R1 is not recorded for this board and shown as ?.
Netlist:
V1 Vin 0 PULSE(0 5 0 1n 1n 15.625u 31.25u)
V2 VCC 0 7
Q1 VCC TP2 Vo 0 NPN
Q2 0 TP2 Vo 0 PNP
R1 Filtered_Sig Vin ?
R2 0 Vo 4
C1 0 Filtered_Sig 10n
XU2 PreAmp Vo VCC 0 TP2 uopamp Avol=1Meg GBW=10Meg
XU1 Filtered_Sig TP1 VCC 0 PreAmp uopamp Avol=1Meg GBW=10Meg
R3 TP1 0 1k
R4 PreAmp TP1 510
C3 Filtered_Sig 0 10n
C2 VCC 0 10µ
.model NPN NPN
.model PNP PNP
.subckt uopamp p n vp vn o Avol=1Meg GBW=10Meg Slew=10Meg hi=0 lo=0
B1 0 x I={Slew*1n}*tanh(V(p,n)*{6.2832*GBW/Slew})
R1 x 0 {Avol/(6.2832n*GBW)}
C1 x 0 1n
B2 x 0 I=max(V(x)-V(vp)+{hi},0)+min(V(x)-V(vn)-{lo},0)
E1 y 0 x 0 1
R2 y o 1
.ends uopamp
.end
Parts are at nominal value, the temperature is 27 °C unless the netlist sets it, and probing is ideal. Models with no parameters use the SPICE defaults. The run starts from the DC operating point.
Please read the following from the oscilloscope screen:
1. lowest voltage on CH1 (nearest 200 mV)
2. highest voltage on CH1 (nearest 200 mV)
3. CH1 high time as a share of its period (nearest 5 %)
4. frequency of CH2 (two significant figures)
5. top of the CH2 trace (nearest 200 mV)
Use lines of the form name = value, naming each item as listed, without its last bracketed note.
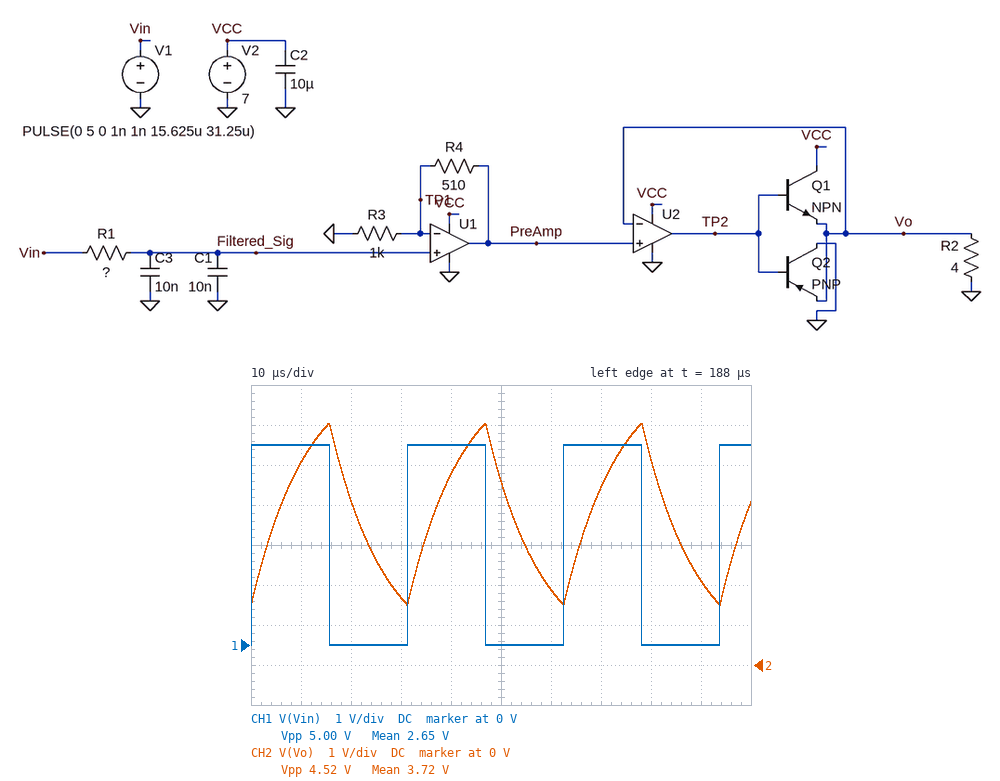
lowest voltage on CH1 = 0 V
highest voltage on CH1 = 5.0 V
CH1 high time as a share of its period = 50 %
frequency of CH2 = 32 kHz
top of the CH2 trace = 6.0 V
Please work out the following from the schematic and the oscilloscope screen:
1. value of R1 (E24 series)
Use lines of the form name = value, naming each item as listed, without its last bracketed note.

value of R1 = 560 Ω
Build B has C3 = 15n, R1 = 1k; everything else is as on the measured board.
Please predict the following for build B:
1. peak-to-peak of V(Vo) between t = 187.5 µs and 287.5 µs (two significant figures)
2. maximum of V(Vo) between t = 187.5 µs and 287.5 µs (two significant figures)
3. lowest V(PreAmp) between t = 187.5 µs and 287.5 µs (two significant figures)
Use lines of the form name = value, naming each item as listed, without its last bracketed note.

peak-to-peak of V(Vo) between t = 187.5 µs and 287.5 µs = 2.3 V
maximum of V(Vo) between t = 187.5 µs and 287.5 µs = 4.9 V
lowest V(PreAmp) between t = 187.5 µs and 287.5 µs = 2.6 V
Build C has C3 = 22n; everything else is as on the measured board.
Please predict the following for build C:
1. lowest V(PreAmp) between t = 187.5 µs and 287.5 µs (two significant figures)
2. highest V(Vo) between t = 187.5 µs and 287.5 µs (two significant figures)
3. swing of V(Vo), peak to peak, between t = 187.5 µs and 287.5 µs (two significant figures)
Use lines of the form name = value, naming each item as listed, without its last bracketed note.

lowest V(PreAmp) between t = 187.5 µs and 287.5 µs = 2.2 V
highest V(Vo) between t = 187.5 µs and 287.5 µs = 5.3 V
swing of V(Vo), peak to peak, between t = 187.5 µs and 287.5 µs = 3.1 V
